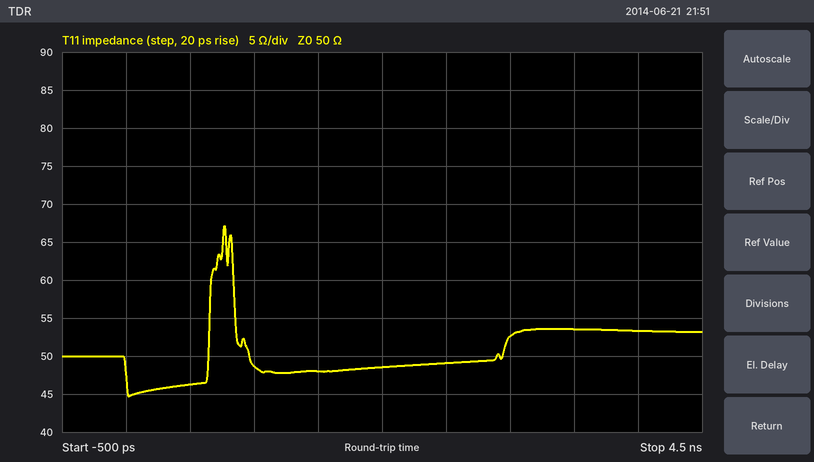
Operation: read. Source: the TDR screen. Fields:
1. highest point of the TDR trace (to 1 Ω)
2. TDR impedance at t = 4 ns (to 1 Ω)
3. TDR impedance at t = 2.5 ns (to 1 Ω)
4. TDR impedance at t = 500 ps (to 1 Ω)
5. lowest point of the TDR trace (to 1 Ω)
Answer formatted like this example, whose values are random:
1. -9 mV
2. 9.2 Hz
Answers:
1. 67 Ω
2. 53 Ω
3. 49 Ω
4. 46 Ω
5. 45 Ω
